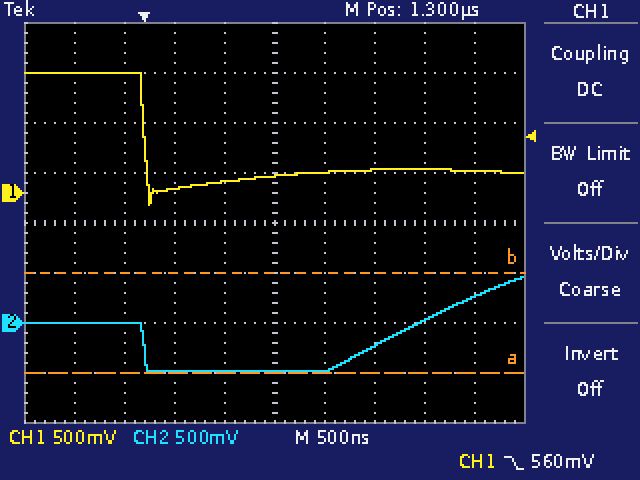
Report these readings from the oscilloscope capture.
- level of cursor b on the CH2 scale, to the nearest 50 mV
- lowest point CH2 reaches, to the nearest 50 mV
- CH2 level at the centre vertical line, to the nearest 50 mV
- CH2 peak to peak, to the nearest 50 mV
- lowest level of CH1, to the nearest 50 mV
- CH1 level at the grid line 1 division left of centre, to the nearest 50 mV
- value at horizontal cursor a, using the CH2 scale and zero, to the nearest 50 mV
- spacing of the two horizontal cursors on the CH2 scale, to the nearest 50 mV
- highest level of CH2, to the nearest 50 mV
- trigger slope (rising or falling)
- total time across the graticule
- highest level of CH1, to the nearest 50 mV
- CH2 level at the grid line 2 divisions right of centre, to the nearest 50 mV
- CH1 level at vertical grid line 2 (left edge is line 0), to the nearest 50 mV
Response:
500 mV
-500 mV
-500 mV
950 mV
-100 mV
100 mV
-500 mV
1.00 V
450 mV
falling
5 µs
1.20 V
-250 mV
1.20 V
